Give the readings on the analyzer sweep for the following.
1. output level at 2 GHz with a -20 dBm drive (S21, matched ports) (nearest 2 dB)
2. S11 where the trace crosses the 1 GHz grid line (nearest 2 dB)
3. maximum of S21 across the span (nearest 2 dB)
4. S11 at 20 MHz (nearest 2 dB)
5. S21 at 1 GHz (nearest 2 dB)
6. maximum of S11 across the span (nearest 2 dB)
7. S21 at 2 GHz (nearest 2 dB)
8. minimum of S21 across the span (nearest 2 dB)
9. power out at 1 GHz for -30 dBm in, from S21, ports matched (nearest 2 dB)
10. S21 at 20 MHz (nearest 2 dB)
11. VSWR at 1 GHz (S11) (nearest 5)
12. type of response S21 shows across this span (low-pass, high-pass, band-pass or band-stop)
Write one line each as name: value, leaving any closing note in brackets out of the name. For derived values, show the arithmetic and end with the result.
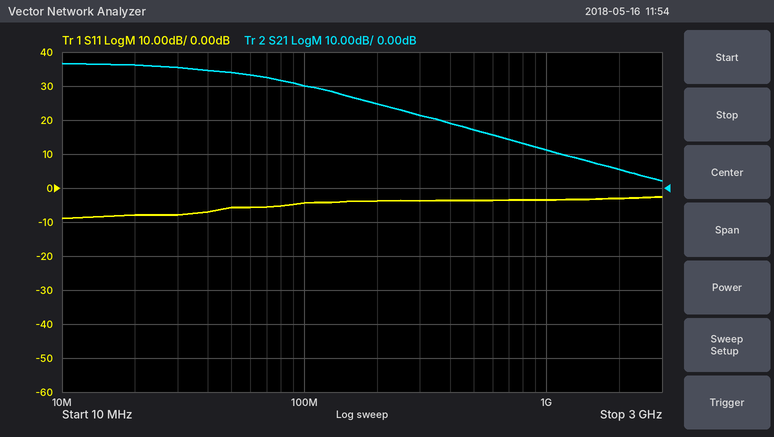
output level at 2 GHz with a -20 dBm drive (S21, matched ports): -20 dBm + (6 dB) = -14 dBm
S11 where the trace crosses the 1 GHz grid line: -4 dB
maximum of S21 across the span: 36 dB
S11 at 20 MHz: -8 dB
S21 at 1 GHz: 12 dB
maximum of S11 across the span: -2 dB
S21 at 2 GHz: 6 dB
minimum of S21 across the span: 2 dB
power out at 1 GHz for -30 dBm in, from S21, ports matched: -30 dBm + (12 dB) = -18 dBm
S21 at 20 MHz: 36 dB
VSWR at 1 GHz (S11): |Γ| = 10^(-4/20) = 0.6310; VSWR = (1 + 0.6310)/(1 − 0.6310) ≈ 4.42, so 5 to the nearest 5
type of response S21 shows across this span: low-pass
